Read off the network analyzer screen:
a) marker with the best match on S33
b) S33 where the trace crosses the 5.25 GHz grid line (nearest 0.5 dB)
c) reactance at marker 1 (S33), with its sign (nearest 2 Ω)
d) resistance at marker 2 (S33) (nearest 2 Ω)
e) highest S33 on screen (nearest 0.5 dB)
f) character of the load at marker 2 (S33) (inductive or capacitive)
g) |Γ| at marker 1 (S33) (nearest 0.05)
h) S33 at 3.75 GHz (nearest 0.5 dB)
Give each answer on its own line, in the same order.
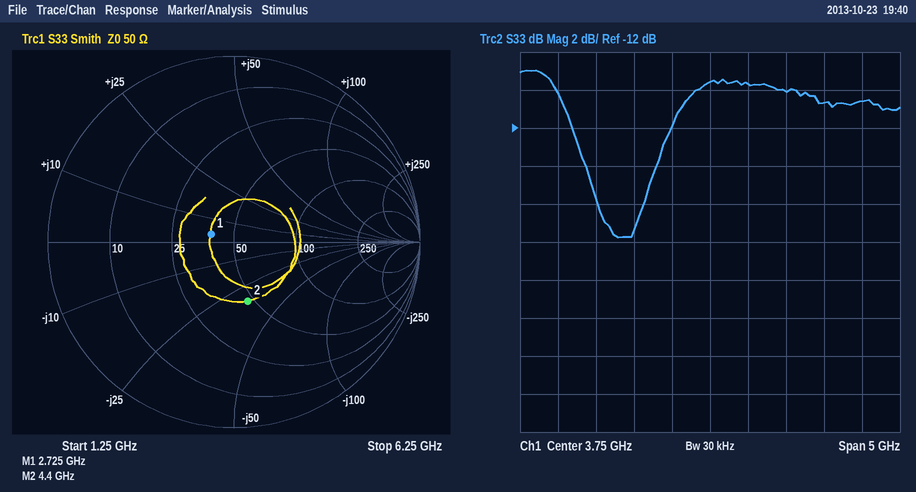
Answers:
marker 1
-10.5 dB
+4 Ω
46 Ω
-9.0 dB
capacitive
0.15
-9.5 dB
